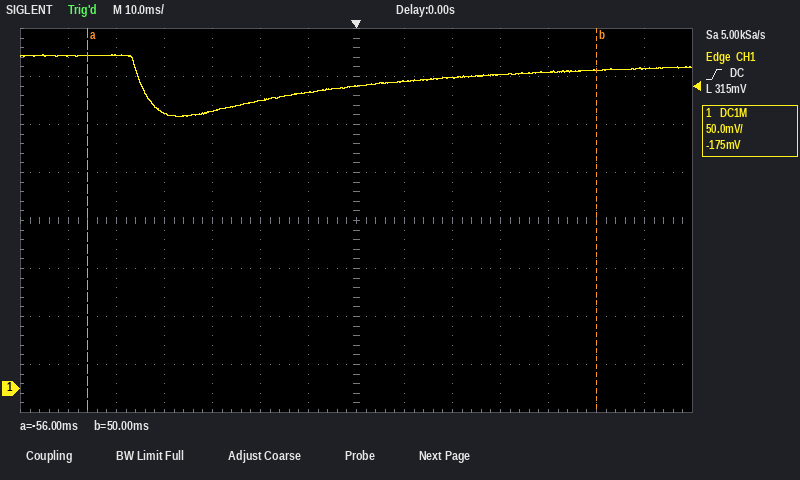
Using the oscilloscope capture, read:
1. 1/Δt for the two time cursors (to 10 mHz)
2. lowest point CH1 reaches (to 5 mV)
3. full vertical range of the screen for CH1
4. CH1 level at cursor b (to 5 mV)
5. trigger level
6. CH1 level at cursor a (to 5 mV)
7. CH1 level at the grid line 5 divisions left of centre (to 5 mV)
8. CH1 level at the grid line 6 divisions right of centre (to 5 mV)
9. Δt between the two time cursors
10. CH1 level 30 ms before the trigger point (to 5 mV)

9.43 Hz
285 mV
400 mV
330 mV
315 mV
345 mV
345 mV
335 mV
106 ms
290 mV
